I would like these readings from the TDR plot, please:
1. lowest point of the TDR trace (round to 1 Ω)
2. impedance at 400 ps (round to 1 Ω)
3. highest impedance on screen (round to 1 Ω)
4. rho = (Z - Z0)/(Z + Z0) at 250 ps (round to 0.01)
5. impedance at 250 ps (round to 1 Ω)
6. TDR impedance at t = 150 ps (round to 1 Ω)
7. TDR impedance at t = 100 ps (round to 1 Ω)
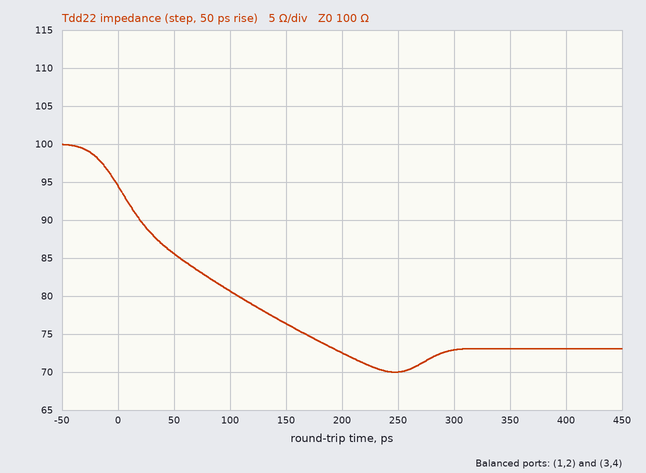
70 Ω
73 Ω
100 Ω
-0.18
70 Ω
76 Ω
81 Ω
